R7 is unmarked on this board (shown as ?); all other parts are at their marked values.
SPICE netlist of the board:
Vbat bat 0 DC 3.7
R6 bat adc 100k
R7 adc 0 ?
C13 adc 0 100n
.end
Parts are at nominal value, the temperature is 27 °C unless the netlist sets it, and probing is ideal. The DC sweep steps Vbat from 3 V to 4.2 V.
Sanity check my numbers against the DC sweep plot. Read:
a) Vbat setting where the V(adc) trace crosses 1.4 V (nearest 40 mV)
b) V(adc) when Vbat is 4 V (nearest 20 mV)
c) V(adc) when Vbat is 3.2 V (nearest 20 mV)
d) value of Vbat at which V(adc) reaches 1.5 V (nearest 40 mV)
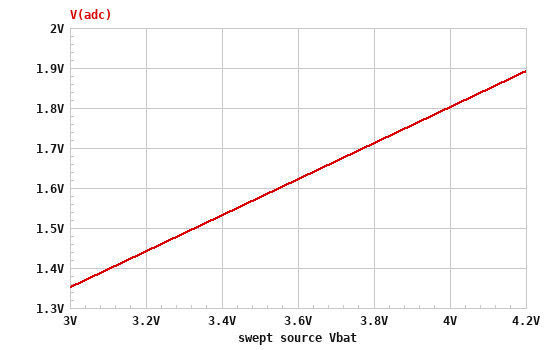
3.12 V
1.80 V
1.44 V
3.32 V
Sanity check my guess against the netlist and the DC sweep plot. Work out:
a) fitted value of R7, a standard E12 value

82 kΩ
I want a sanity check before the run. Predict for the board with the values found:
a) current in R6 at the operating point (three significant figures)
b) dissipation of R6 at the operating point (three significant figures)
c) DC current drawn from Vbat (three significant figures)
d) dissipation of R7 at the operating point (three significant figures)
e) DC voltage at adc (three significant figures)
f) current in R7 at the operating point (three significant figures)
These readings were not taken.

20.3 µA
41.3 µW
20.3 µA
33.9 µW
1.67 V
20.3 µA
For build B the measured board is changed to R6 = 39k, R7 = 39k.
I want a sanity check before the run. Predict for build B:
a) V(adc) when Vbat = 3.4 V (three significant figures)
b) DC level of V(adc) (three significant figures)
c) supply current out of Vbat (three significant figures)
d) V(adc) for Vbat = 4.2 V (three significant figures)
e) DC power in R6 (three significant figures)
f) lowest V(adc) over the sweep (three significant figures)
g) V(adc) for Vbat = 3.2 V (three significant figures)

1.70 V
1.85 V
47.4 µA
2.10 V
87.8 µW
1.50 V
1.60 V
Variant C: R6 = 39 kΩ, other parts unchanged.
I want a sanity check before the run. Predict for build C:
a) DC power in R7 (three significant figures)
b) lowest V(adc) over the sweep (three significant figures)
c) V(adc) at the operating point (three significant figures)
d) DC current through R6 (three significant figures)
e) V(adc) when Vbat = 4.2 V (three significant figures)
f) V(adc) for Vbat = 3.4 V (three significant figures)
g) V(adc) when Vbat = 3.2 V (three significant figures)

76.7 µW
2.03 V
2.51 V
30.6 µA
2.85 V
2.30 V
2.17 V
